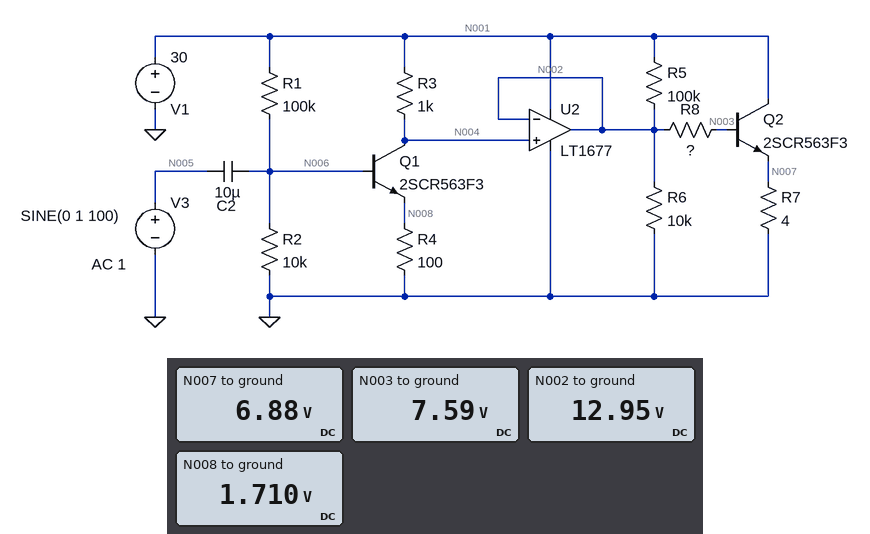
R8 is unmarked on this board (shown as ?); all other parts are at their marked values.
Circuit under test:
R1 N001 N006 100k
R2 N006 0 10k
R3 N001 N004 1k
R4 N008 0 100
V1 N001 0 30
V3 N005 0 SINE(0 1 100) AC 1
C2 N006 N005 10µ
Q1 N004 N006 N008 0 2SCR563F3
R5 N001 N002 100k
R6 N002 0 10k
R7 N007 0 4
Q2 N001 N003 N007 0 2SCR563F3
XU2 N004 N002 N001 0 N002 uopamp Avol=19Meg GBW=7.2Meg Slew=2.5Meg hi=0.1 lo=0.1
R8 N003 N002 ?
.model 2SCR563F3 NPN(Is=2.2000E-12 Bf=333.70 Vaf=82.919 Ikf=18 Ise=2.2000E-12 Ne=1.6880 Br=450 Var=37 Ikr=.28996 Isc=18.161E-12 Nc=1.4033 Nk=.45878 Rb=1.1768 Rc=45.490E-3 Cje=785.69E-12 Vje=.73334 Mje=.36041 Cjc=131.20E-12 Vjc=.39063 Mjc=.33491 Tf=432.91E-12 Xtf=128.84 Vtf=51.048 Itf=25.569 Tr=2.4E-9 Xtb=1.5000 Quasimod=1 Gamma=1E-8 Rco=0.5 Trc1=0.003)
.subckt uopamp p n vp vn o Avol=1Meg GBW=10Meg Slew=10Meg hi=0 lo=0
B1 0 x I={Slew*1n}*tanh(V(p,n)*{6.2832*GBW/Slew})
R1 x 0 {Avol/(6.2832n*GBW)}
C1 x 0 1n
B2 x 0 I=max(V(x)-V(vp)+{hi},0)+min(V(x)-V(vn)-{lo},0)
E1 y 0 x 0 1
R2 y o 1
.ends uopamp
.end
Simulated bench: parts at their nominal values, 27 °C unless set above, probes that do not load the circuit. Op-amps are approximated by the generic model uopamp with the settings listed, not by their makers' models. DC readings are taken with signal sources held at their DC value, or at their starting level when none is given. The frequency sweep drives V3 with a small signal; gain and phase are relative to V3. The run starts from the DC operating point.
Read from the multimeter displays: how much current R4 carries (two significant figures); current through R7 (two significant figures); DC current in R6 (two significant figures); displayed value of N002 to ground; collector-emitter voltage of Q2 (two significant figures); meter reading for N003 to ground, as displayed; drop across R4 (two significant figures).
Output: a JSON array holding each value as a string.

["17 mA", "1.7 A", "1.3 mA", "12.95 V", "23 V", "7.59 V", "1.7 V"]
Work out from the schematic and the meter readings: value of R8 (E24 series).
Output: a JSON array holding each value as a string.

["1.2 kΩ"]
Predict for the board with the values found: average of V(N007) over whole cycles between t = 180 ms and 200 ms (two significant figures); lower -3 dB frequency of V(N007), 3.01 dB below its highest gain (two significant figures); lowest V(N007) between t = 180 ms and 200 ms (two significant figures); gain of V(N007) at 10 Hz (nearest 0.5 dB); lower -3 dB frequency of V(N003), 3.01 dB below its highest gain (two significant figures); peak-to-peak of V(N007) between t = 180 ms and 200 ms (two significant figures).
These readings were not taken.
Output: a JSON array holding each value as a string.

["6.8 V", "2.3 Hz", "1.5 V", "14.0 dB", "2.3 Hz", "10 V"]
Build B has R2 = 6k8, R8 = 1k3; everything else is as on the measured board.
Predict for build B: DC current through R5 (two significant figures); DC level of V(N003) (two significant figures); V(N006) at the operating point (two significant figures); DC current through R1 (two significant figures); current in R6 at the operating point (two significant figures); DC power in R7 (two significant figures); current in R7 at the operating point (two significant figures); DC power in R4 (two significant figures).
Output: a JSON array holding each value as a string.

["110 µA", "10 V", "1.7 V", "280 µA", "1.9 mA", "22 W", "2.4 A", "13 mW"]
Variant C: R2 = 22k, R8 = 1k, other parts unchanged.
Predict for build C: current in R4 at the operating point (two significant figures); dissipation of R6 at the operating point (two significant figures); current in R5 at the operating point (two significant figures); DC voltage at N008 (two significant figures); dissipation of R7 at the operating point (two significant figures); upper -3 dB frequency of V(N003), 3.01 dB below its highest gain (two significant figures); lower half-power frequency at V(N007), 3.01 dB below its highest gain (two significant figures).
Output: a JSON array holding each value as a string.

["27 mA", "800 µW", "270 µA", "2.7 V", "470 mW", "740 kHz", "66 Hz"]
